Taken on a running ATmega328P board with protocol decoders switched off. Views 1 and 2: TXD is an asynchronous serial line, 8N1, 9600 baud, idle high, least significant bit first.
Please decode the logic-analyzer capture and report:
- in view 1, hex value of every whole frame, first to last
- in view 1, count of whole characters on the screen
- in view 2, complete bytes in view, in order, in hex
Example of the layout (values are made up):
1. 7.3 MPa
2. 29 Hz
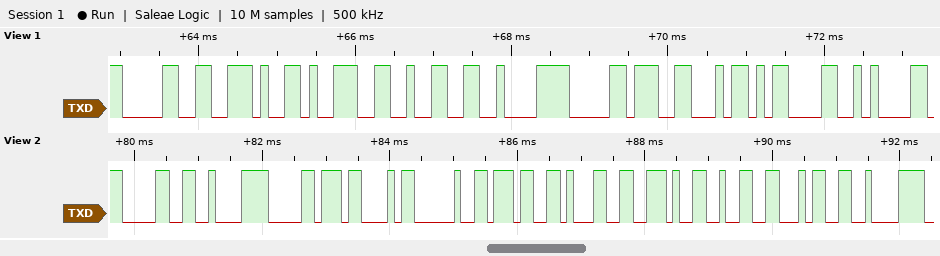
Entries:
1. 30 2E 39 32 C2 B0 46 0D 0A
2. 9
3. 0x30 0xC2 0xB0 0x43 0x20 0x37 0x31 0x2E 0x32 0x34 0xC2
